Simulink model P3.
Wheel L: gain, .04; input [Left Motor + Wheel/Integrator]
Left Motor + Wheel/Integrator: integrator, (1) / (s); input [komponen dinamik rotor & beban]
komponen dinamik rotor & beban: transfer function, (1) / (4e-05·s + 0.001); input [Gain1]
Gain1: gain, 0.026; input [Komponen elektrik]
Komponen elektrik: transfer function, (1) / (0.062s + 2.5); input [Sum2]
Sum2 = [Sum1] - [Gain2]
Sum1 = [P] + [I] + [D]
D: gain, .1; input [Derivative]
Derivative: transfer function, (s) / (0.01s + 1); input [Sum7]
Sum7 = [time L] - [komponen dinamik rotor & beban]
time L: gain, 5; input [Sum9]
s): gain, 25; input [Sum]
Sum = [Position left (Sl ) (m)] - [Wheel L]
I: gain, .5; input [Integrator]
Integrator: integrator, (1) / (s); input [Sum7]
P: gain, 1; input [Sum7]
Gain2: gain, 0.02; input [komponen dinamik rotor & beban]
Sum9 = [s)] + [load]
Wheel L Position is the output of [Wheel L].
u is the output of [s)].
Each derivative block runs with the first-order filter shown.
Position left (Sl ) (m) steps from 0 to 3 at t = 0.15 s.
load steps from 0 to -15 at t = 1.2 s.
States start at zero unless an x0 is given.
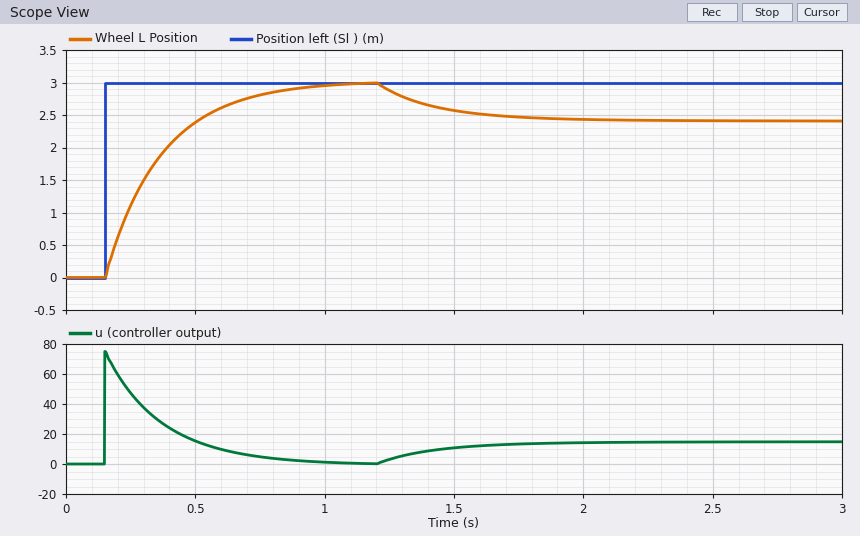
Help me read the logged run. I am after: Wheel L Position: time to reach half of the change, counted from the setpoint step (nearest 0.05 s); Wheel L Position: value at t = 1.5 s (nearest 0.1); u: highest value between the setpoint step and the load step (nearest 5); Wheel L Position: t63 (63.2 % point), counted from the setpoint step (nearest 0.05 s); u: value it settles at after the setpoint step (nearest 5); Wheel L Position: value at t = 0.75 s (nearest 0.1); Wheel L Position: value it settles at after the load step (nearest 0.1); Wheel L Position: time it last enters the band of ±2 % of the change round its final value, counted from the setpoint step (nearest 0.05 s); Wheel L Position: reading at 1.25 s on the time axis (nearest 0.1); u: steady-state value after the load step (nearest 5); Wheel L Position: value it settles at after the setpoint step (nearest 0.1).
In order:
0.15 s
2.6
75
0.20 s
0
2.8
2.4
0.80 s
2.9
15
3.0
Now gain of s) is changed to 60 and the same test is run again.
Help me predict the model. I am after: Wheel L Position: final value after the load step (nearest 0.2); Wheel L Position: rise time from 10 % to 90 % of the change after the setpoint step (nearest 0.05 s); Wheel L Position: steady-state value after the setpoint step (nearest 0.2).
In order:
2.8
0.20 s
3.0
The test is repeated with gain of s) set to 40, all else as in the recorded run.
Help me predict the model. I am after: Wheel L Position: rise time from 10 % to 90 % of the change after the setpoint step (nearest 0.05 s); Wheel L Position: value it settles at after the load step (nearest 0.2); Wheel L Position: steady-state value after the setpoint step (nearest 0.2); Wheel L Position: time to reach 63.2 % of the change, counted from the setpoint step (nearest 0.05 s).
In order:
0.30 s
2.6
3.0
0.15 s
